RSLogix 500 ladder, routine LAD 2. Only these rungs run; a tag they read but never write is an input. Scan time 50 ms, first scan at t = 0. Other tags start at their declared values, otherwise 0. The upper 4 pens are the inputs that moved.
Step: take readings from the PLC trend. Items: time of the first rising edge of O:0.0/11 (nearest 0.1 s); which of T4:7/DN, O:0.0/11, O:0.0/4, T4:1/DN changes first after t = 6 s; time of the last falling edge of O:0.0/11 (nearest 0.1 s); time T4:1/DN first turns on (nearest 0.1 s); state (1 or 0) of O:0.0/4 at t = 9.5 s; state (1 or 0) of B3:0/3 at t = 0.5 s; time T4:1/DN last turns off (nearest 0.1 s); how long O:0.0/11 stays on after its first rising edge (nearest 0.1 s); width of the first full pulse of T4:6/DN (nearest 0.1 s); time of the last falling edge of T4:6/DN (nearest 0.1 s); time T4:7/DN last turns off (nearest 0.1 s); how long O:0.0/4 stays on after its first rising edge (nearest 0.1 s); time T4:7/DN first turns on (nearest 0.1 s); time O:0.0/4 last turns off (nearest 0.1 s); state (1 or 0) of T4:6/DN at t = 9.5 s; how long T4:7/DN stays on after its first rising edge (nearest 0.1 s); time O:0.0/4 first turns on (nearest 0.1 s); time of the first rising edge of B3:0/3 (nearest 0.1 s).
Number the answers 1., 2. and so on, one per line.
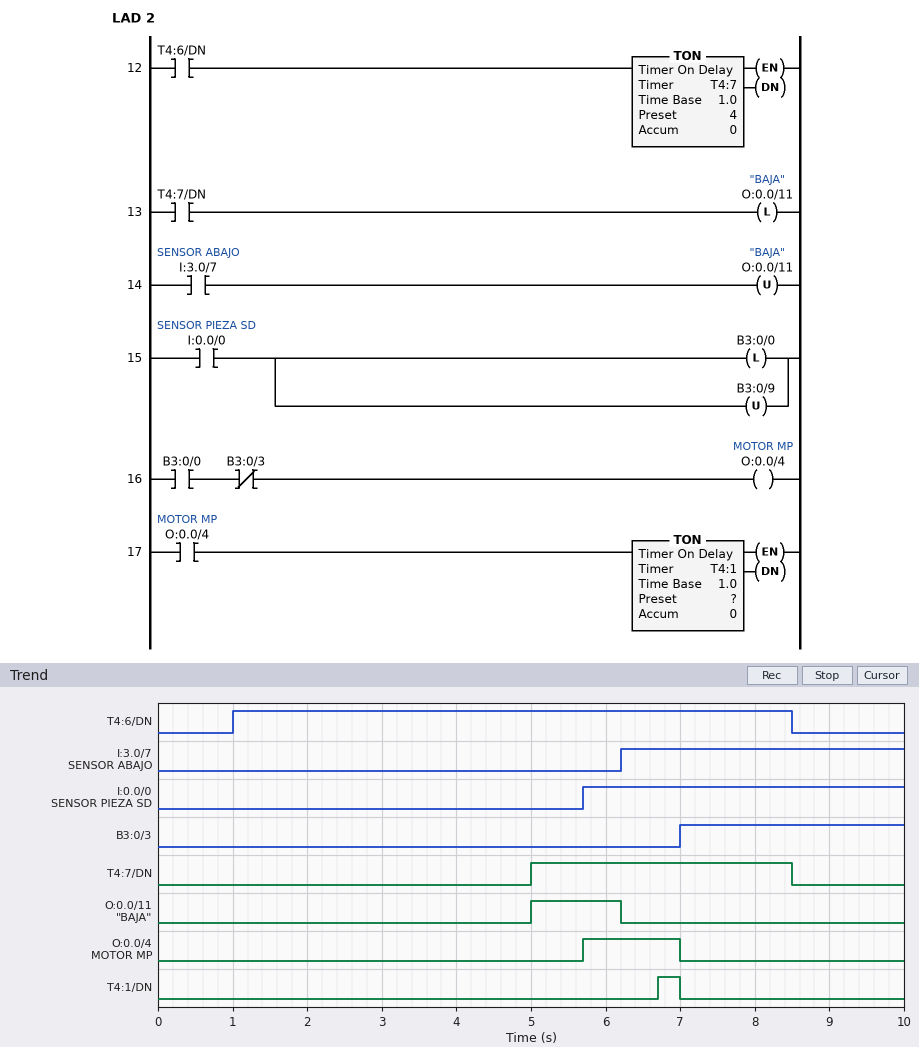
1. 5.0 s
2. O:0.0/11
3. 6.2 s
4. 6.7 s
5. 0
6. 0
7. 7.0 s
8. 1.2 s
9. 7.5 s
10. 8.5 s
11. 8.5 s
12. 1.3 s
13. 5.0 s
14. 7.0 s
15. 0
16. 3.5 s
17. 5.7 s
18. 7.0 s
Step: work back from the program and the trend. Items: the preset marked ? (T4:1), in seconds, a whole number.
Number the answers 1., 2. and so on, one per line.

1. 1 s
